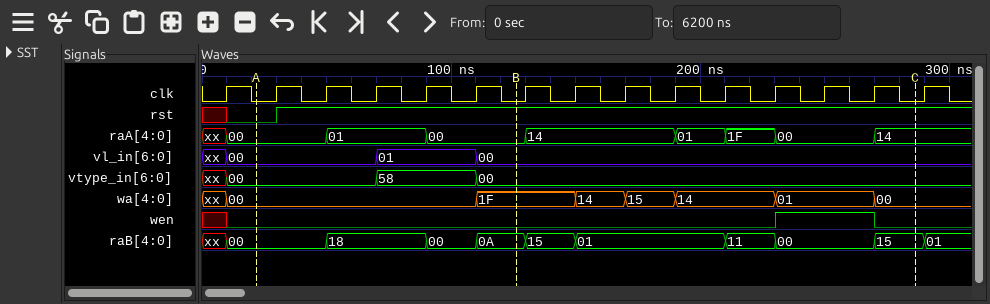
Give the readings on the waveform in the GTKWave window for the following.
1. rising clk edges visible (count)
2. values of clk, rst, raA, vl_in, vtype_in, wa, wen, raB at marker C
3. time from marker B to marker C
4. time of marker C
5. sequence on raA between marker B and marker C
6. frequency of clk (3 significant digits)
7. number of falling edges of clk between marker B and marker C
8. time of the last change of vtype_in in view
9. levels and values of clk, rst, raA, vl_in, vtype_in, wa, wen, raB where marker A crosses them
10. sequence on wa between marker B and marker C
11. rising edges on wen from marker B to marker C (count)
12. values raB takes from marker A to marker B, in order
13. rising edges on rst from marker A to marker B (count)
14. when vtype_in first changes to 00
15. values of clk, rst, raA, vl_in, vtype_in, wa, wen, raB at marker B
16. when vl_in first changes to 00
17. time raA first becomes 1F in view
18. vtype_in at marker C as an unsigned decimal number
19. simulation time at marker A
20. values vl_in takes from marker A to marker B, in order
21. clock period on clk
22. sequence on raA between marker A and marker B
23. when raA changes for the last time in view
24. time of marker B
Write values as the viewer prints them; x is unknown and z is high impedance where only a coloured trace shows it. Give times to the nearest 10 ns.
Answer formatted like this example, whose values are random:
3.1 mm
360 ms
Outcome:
15
clk=0, rst=1, raA=14, vl_in=00, vtype_in=00, wa=00, wen=0, raB=15
160 ns
290 ns
00, 14, 01, 1F, 00, 14
50.0 MHz
8
110 ns
clk=0, rst=0, raA=00, vl_in=00, vtype_in=00, wa=00, wen=0, raB=00
1F, 14, 15, 14, 01, 00
1
00, 18, 00, 0A
1
10 ns
clk=0, rst=1, raA=00, vl_in=00, vtype_in=00, wa=1F, wen=0, raB=0A
10 ns
210 ns
0
20 ns
00, 01, 00
20 ns
00, 01, 00
270 ns
130 ns
